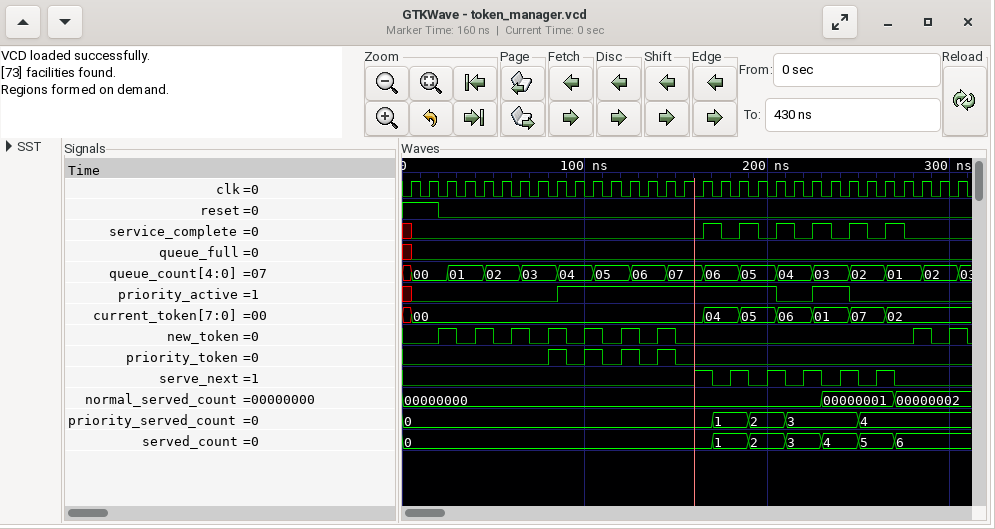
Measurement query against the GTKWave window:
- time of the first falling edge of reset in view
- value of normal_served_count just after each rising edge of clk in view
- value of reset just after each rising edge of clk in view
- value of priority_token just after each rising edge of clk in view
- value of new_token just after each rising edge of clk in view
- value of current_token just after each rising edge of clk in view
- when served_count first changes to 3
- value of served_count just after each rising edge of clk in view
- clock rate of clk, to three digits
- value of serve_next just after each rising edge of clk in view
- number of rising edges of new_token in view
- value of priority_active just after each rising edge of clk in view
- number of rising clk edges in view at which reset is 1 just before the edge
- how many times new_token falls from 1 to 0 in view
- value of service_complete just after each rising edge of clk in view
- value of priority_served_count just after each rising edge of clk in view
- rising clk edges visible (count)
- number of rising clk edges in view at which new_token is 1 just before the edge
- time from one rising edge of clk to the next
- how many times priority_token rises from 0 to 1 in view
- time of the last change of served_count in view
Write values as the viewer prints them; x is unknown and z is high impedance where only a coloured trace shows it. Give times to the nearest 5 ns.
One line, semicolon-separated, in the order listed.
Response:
20 ns; 00000000, 00000000, 00000000, 00000000, 00000000, 00000000, 00000000, 00000000, 00000000, 00000000, 00000000, 00000000, 00000000, 00000000, 00000000, 00000000, 00000000, 00000000, 00000000, 00000000, 00000000, 00000000, 00000000, 00000001, 00000001, 00000001, 00000001, 00000002, 00000002, 00000002, 00000002; 1 1 0 0 0 0 0 0 0 0 0 0 0 0 0 0 0 0 0 0 0 0 0 0 0 0 0 0 0 0 0; 0 0 0 0 0 0 0 0 1 0 1 0 1 0 1 0 0 0 0 0 0 0 0 0 0 0 0 0 0 0 0; 0 0 1 0 1 0 1 0 1 0 1 0 1 0 1 0 0 0 0 0 0 0 0 0 0 0 0 0 1 0 1; 00, 00, 00, 00, 00, 00, 00, 00, 00, 00, 00, 00, 00, 00, 00, 00, 04, 04, 05, 05, 06, 06, 01, 01, 07, 07, 02, 02, 02, 02, 02; 210 ns; 0, 0, 0, 0, 0, 0, 0, 0, 0, 0, 0, 0, 0, 0, 0, 0, 0, 1, 1, 2, 2, 3, 3, 4, 4, 5, 5, 6, 6, 6, 6; 100 MHz; 0 0 0 0 0 0 0 0 0 0 0 0 0 0 0 0 1 0 1 0 1 0 1 0 1 0 1 0 0 0 0; 9; 0 0 0 0 0 0 0 0 1 1 1 1 1 1 1 1 1 1 1 1 0 0 1 1 0 0 0 0 0 0 0; 2; 9; 0 0 0 0 0 0 0 0 0 0 0 0 0 0 0 0 1 0 1 0 1 0 1 0 1 0 1 0 0 0 0; 0, 0, 0, 0, 0, 0, 0, 0, 0, 0, 0, 0, 0, 0, 0, 0, 0, 1, 1, 2, 2, 3, 3, 3, 3, 4, 4, 4, 4, 4, 4; 31; 9; 10 ns; 4; 270 ns
